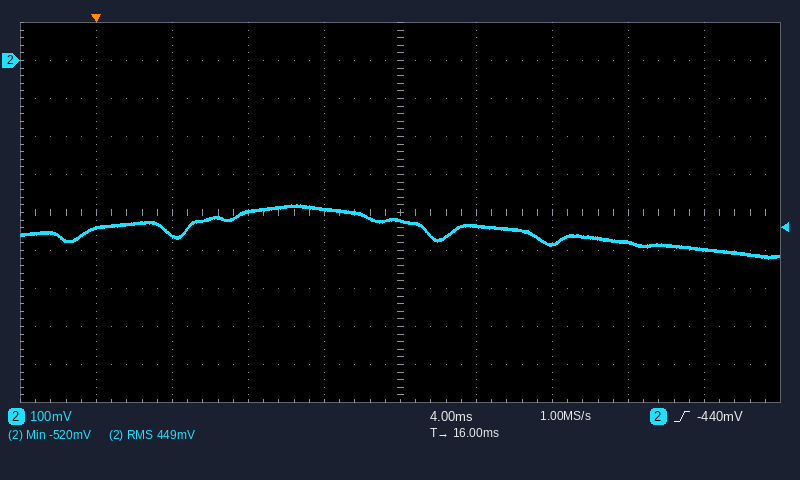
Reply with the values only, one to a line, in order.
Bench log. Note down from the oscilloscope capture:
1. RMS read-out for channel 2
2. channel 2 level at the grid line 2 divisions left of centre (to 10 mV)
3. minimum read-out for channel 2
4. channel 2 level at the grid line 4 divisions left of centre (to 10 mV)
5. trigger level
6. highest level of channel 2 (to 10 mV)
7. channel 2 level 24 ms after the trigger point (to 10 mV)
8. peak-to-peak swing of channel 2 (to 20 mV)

449 mV
-400 mV
-520 mV
-440 mV
-440 mV
-380 mV
-480 mV
140 mV
